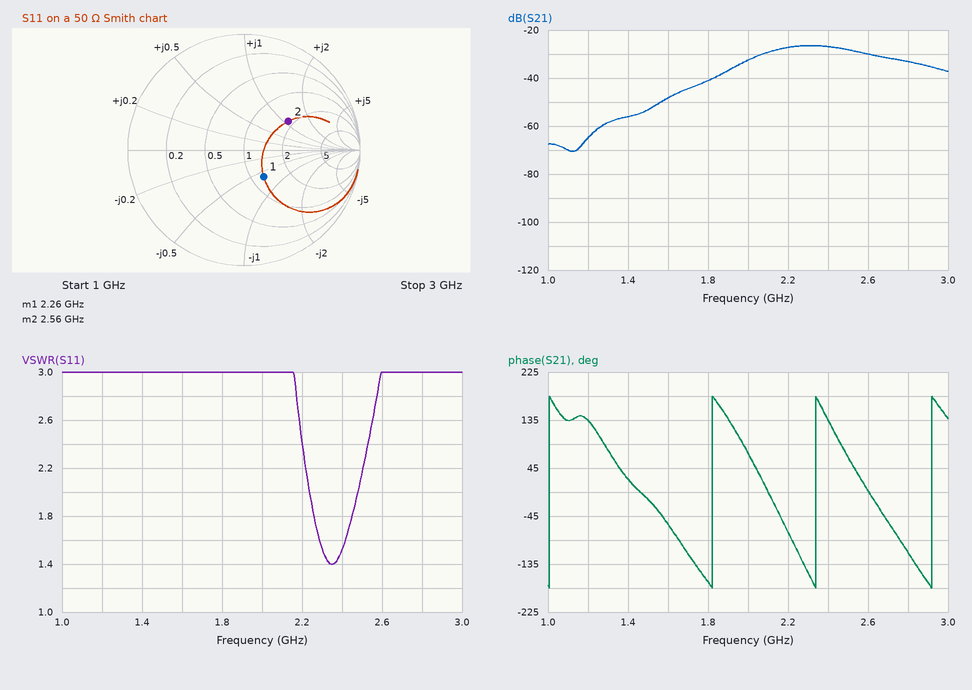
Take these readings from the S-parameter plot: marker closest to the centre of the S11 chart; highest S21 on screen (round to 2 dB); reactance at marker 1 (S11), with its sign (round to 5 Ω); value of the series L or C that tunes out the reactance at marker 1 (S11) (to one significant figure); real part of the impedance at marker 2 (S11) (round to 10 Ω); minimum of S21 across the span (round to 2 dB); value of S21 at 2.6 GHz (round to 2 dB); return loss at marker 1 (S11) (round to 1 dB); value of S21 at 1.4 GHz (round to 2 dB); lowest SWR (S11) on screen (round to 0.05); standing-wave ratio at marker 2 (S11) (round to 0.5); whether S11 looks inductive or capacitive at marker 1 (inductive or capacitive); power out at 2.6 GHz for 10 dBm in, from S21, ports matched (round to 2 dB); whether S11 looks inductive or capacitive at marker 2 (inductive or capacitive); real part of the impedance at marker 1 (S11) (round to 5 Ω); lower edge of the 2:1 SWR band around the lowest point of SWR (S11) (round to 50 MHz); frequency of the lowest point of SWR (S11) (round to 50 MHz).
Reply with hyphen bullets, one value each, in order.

- marker 1
- -26 dB
- -30 Ω
- 2 nH
- 90 Ω
- -70 dB
- -30 dB
- 11 dB
- -56 dB
- 1.40
- 2.5
- capacitive
- -20 dBm
- inductive
- 60 Ω
- 2.25 GHz
- 2.35 GHz
